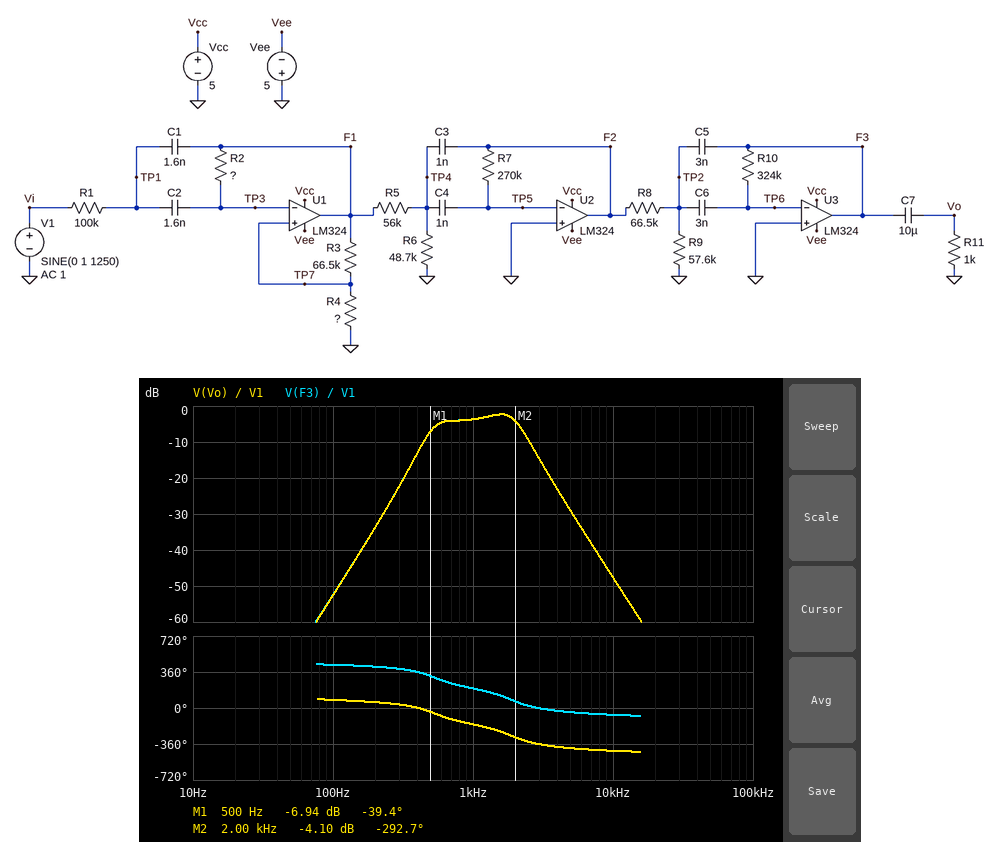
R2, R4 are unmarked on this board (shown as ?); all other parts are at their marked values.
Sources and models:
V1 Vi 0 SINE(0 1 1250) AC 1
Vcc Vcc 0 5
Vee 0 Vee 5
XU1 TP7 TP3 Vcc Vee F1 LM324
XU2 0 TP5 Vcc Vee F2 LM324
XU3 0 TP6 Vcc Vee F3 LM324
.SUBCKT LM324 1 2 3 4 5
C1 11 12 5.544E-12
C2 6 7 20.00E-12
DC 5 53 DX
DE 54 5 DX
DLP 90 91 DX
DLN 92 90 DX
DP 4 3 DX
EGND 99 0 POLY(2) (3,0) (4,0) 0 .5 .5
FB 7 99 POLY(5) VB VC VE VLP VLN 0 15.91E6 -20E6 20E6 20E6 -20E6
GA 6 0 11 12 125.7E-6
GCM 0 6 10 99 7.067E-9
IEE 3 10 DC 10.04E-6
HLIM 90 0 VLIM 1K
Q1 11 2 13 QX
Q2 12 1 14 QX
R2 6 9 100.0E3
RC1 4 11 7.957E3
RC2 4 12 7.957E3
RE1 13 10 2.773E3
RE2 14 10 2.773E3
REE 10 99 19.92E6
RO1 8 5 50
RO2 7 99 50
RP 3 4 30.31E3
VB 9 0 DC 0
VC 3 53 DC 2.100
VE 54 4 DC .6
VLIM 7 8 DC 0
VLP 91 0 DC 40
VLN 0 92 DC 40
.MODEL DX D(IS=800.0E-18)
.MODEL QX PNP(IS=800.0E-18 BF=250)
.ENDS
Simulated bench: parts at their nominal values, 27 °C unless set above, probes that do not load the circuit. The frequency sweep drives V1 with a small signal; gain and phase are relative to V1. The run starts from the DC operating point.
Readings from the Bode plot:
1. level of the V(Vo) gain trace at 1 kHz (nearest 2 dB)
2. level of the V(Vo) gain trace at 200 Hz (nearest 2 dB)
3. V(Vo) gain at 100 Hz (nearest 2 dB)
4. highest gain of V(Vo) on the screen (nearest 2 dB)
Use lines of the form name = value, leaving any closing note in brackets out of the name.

level of the V(Vo) gain trace at 1 kHz = -4 dB
level of the V(Vo) gain trace at 200 Hz = -34 dB
V(Vo) gain at 100 Hz = -52 dB
highest gain of V(Vo) on the screen = -2 dB
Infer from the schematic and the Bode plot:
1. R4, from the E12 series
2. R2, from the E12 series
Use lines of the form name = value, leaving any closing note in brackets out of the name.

R4, from the E12 series = 56 kΩ
R2, from the E12 series = 56 kΩ
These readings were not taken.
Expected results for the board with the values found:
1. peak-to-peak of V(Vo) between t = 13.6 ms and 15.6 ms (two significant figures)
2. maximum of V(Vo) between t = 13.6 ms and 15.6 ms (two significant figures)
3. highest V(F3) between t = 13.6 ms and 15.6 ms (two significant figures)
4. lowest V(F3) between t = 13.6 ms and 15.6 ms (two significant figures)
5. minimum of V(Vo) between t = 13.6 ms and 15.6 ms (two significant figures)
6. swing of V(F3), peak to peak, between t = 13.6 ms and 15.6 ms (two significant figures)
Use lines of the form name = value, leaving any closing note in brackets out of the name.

peak-to-peak of V(Vo) between t = 13.6 ms and 15.6 ms = 1.4 V
maximum of V(Vo) between t = 13.6 ms and 15.6 ms = 710 mV
highest V(F3) between t = 13.6 ms and 15.6 ms = 700 mV
lowest V(F3) between t = 13.6 ms and 15.6 ms = -710 mV
minimum of V(Vo) between t = 13.6 ms and 15.6 ms = -710 mV
swing of V(F3), peak to peak, between t = 13.6 ms and 15.6 ms = 1.4 V
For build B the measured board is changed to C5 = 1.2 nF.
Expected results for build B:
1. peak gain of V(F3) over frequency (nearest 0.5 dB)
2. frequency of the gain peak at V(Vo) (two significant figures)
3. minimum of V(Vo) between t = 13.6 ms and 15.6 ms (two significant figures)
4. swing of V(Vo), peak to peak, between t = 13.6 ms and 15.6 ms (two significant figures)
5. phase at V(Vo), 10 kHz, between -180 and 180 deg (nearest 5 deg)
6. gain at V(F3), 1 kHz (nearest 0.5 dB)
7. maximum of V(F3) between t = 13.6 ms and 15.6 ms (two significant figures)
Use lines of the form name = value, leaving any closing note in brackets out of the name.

peak gain of V(F3) over frequency = 6.5 dB
frequency of the gain peak at V(Vo) = 1.5 kHz
minimum of V(Vo) between t = 13.6 ms and 15.6 ms = -2.1 V
swing of V(Vo), peak to peak, between t = 13.6 ms and 15.6 ms = 4.2 V
phase at V(Vo), 10 kHz, between -180 and 180 deg = -65 deg
gain at V(F3), 1 kHz = 6.0 dB
maximum of V(F3) between t = 13.6 ms and 15.6 ms = 2.1 V
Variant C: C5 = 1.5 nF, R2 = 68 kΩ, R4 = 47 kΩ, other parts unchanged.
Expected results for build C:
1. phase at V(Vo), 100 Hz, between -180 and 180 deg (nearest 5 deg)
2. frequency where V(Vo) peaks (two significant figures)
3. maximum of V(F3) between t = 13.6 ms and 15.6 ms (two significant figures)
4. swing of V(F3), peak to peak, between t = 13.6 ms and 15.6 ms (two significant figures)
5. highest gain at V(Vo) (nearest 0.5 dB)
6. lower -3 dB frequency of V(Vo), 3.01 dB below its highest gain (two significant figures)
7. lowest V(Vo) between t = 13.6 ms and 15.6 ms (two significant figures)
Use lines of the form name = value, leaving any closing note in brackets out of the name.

phase at V(Vo), 100 Hz, between -180 and 180 deg = 85 deg
frequency where V(Vo) peaks = 1.5 kHz
maximum of V(F3) between t = 13.6 ms and 15.6 ms = 1.8 V
swing of V(F3), peak to peak, between t = 13.6 ms and 15.6 ms = 3.7 V
highest gain at V(Vo) = 5.5 dB
lower -3 dB frequency of V(Vo), 3.01 dB below its highest gain = 710 Hz
lowest V(Vo) between t = 13.6 ms and 15.6 ms = -1.8 V
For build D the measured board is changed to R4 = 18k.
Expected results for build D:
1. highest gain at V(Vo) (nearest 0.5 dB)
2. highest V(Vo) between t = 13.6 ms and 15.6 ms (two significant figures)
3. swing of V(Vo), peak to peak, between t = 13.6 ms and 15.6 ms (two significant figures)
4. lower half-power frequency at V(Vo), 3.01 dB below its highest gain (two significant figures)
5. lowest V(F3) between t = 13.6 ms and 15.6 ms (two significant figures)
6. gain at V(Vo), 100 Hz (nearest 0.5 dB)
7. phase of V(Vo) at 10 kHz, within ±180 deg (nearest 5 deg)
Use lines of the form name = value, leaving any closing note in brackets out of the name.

highest gain at V(Vo) = -7.0 dB
highest V(Vo) between t = 13.6 ms and 15.6 ms = 400 mV
swing of V(Vo), peak to peak, between t = 13.6 ms and 15.6 ms = 810 mV
lower half-power frequency at V(Vo), 3.01 dB below its highest gain = 520 Hz
lowest V(F3) between t = 13.6 ms and 15.6 ms = -410 mV
gain at V(Vo), 100 Hz = -56.0 dB
phase of V(Vo) at 10 kHz, within ±180 deg = -65 deg
